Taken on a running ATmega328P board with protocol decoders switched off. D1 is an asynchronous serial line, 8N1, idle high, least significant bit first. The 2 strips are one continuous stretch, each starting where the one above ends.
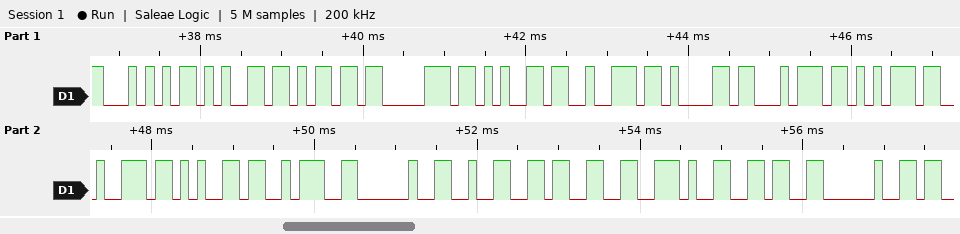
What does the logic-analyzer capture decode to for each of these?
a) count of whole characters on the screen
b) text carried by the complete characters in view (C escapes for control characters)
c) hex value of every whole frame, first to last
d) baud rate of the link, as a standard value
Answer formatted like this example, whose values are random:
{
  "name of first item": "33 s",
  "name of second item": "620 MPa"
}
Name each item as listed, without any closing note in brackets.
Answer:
{
  "count of whole characters on the screen": "18",
  "text carried by the complete characters in view": "\"Temperature: 23.6 \"",
  "hex value of every whole frame, first to last": "54 65 6D 70 65 72 61 74 75 72 65 3A 20 32 33 2E 36 20",
  "baud rate of the link, as a standard value": "9600 baud"
}
